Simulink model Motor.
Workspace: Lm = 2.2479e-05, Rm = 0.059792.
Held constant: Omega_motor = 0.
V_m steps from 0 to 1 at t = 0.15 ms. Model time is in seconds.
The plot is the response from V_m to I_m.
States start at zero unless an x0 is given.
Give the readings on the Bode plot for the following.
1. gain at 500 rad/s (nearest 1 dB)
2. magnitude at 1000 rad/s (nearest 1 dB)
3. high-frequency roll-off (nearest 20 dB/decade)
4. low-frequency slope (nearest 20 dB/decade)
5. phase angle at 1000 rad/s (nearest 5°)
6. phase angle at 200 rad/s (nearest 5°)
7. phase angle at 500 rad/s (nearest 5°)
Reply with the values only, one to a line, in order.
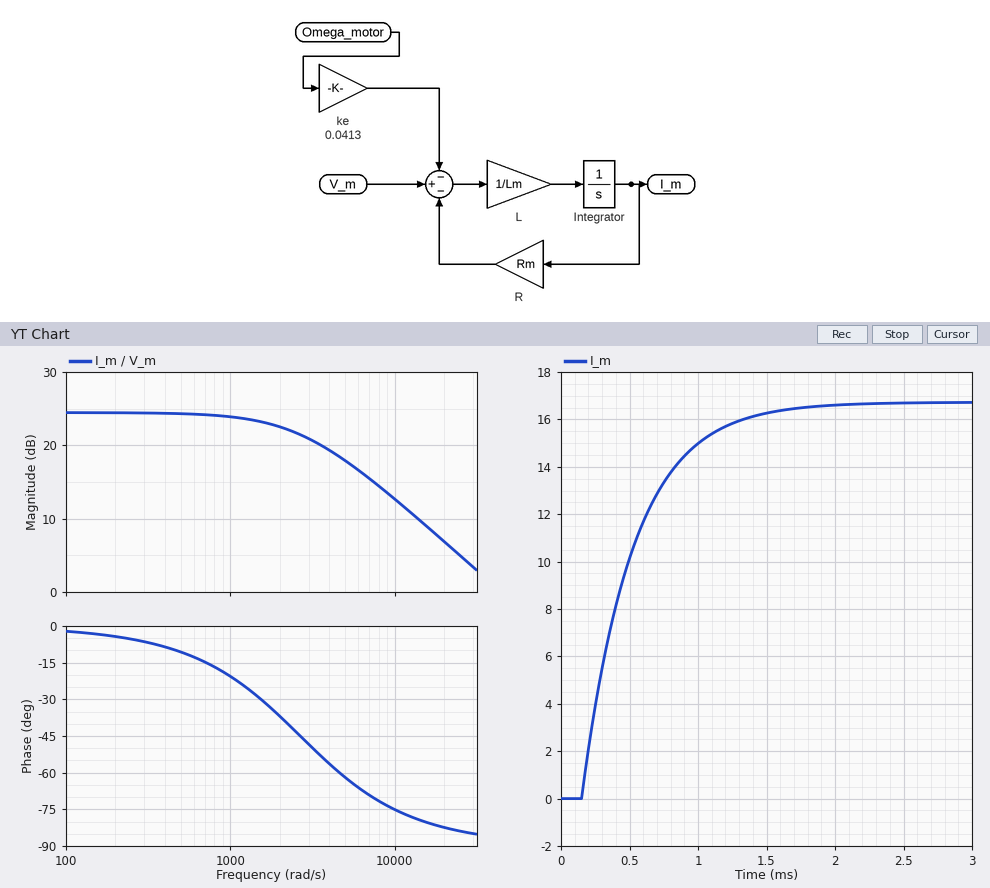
24 dB
24 dB
-20 dB/decade
0 dB/decade
-20°
-5°
-10°
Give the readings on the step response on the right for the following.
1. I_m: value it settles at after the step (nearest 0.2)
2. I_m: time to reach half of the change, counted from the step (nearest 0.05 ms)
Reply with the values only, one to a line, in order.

16.8
0.25 ms
